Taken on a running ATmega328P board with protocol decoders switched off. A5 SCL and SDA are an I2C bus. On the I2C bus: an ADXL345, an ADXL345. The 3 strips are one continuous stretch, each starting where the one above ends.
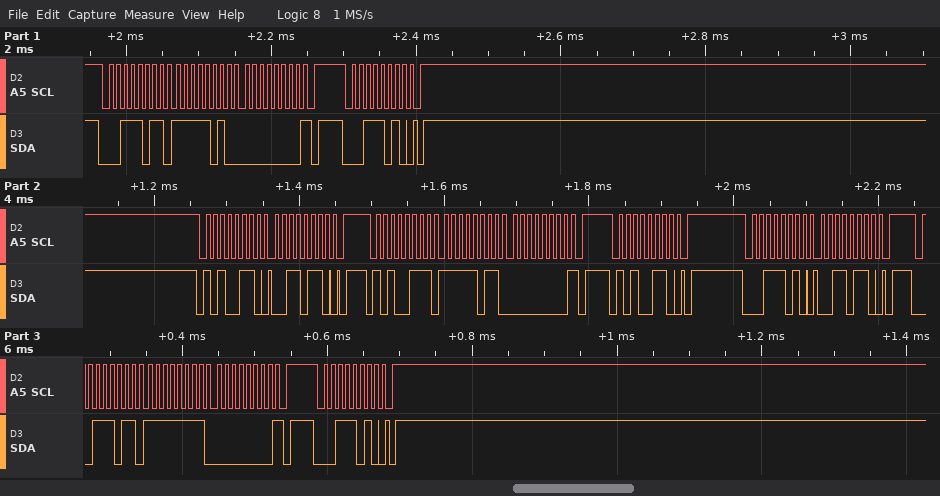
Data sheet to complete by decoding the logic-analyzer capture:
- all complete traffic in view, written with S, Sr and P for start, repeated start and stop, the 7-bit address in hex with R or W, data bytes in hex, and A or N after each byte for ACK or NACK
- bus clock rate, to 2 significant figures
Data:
S 1DR A FA A 00 N P S 1DW A P S 53W A 36 A P S 53R A FB A 00 N P S 53W A P S 1DW A 36 A P S 1DR A FF A 00 N P S 1DW A P
100 kHz
